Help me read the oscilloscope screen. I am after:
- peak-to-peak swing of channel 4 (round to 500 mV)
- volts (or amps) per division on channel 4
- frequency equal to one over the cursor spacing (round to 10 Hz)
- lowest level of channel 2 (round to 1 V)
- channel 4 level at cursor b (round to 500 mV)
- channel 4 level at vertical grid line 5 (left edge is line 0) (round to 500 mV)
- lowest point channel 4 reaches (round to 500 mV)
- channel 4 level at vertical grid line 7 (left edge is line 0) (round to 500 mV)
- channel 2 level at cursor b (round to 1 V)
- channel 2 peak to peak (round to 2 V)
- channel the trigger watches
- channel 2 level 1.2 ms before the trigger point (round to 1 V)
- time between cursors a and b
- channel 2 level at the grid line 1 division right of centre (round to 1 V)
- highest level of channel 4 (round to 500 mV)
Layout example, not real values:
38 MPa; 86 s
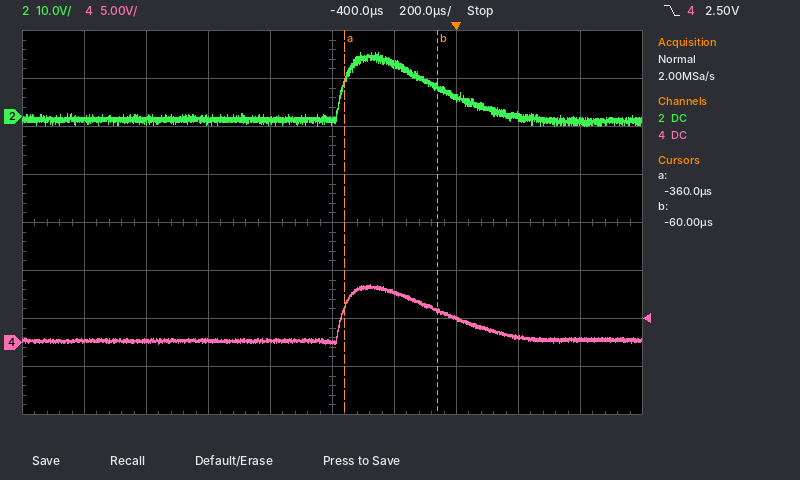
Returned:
6.0 V; 5 V; 3.33 kHz; -2 V; 3.5 V; 0.0 V; 0.0 V; 2.5 V; 6 V; 16 V; channel 4; 0 V; 300 µs; 11 V; 6.0 V
